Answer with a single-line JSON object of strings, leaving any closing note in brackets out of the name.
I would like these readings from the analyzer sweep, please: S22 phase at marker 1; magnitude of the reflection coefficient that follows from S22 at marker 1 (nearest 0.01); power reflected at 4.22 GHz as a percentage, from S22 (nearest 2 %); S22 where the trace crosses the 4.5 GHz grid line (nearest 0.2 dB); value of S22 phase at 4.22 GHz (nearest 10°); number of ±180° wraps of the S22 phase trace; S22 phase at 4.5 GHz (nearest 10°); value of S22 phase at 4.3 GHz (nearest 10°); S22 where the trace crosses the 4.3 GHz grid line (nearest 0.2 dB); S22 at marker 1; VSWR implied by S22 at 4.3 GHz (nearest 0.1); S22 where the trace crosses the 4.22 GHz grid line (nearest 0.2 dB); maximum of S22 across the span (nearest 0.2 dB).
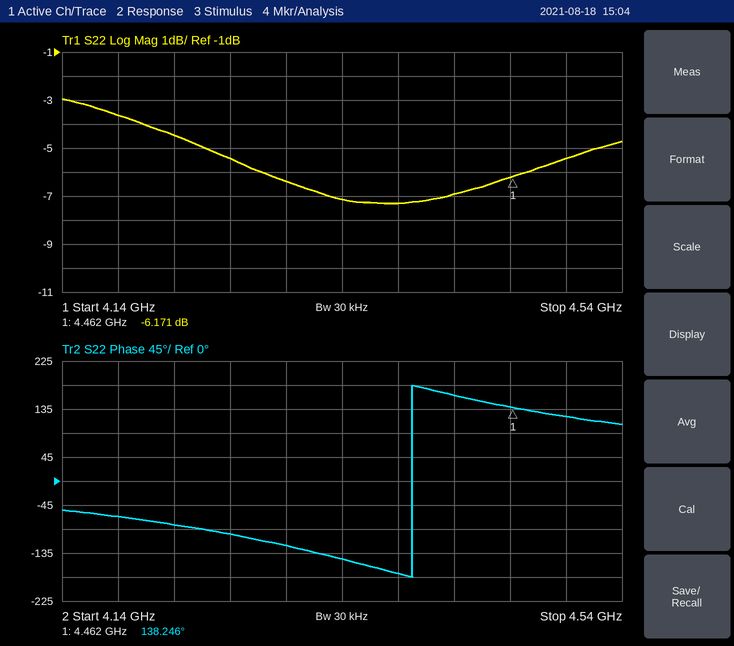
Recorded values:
{"S22 phase at marker 1": "138.246°", "magnitude of the reflection coefficient that follows from S22 at marker 1": "0.49", "power reflected at 4.22 GHz as a percentage, from S22": "36 %", "S22 where the trace crosses the 4.5 GHz grid line": "-5.4 dB", "value of S22 phase at 4.22 GHz": "-80°", "number of ±180° wraps of the S22 phase trace": "1", "S22 phase at 4.5 GHz": "120°", "value of S22 phase at 4.3 GHz": "-120°", "S22 where the trace crosses the 4.3 GHz grid line": "-6.4 dB", "S22 at marker 1": "-6.171 dB", "VSWR implied by S22 at 4.3 GHz": "2.8", "S22 where the trace crosses the 4.22 GHz grid line": "-4.4 dB", "maximum of S22 across the span": "-3.0 dB"}
